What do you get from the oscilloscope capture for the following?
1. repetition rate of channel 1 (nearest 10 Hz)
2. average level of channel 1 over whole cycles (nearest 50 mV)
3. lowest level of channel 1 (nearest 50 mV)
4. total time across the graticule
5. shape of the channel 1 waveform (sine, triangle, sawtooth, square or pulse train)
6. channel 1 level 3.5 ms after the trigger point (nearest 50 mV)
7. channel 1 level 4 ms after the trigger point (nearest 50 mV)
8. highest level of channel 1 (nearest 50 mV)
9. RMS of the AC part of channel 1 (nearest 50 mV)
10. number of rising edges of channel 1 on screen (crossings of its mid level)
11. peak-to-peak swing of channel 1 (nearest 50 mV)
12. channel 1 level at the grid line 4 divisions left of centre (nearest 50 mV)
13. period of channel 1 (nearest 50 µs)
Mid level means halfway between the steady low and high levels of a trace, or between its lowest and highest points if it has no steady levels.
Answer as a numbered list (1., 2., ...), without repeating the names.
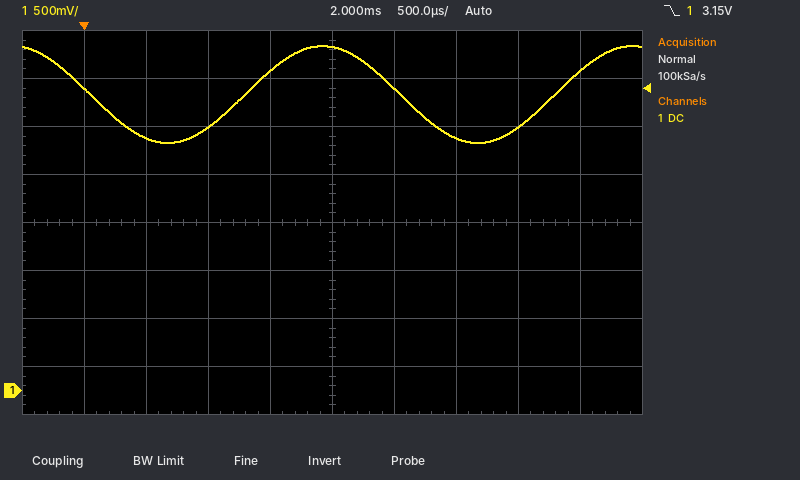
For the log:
1. 400 Hz
2. 3.10 V
3. 2.60 V
4. 5 ms
5. sine
6. 2.75 V
7. 3.35 V
8. 3.60 V
9. 350 mV
10. 2
11. 1.00 V
12. 3.15 V
13. 2.50 ms
